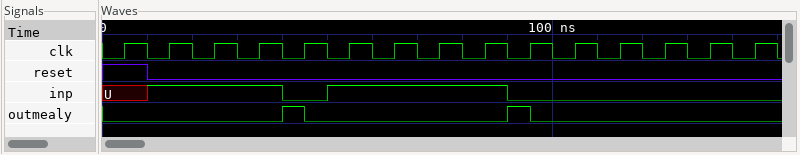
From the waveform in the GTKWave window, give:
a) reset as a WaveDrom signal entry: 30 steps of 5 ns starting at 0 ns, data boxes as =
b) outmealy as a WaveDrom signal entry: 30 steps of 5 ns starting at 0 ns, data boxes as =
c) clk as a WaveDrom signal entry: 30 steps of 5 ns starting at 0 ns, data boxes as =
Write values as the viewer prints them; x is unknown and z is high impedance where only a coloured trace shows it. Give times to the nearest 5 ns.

{name: 'reset', wave: '1.0...........................'}
{name: 'outmealy', wave: '0.......10........10..........'}
{name: 'clk', wave: '010101010101010101010101010101'}
